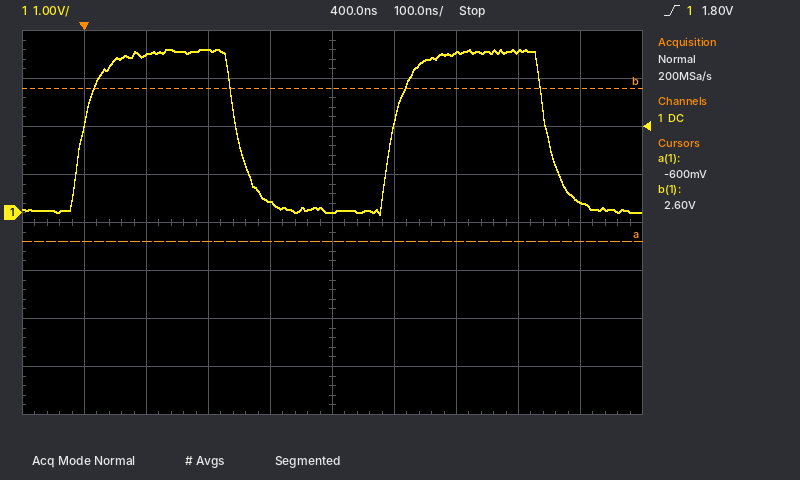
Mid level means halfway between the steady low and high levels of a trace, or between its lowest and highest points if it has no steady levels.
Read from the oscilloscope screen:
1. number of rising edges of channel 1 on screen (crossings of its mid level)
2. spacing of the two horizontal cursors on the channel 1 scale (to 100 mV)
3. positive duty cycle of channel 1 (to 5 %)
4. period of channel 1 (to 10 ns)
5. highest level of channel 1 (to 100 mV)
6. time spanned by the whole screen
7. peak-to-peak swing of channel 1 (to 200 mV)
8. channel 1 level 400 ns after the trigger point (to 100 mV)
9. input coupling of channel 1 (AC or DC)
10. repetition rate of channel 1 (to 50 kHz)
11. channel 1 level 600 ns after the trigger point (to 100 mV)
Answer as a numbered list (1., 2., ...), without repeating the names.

1. 2
2. 3.2 V
3. 50 %
4. 500 ns
5. 3.4 V
6. 1 µs
7. 3.4 V
8. 0.0 V
9. DC
10. 2.00 MHz
11. 3.3 V
